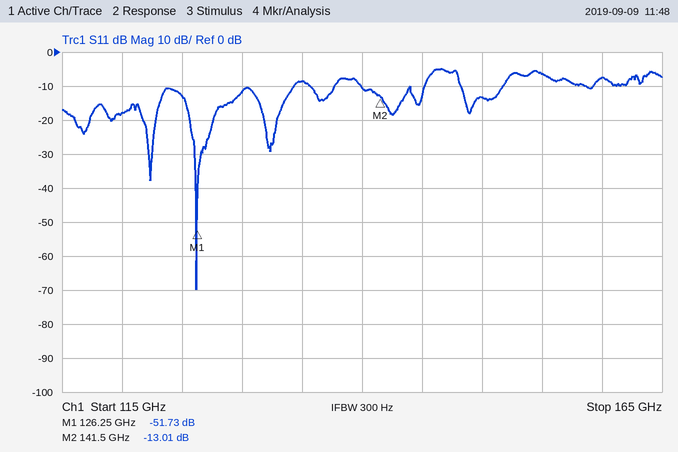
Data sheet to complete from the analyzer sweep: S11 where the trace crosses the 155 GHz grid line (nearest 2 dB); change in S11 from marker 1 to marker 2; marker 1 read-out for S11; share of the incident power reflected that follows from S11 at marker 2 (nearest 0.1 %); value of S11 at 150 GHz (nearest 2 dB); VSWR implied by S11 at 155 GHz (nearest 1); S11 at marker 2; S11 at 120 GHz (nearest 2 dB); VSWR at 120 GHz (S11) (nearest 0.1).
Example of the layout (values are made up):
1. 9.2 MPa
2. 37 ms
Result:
1. -6 dB
2. 38.72 dB
3. -51.73 dB
4. 5.0 %
5. -14 dB
6. 3
7. -13.01 dB
8. -18 dB
9. 1.3
